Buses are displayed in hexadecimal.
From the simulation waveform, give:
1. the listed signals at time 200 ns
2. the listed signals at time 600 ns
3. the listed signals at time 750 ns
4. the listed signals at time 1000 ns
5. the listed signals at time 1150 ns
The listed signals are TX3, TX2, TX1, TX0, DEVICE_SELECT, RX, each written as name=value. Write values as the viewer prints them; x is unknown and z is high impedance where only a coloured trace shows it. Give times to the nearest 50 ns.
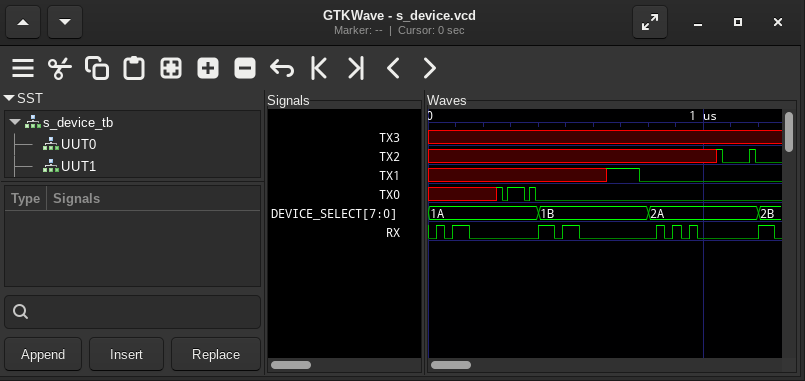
TX3=x, TX2=x, TX1=x, TX0=x, DEVICE_SELECT=1A, RX=0
TX3=x, TX2=x, TX1=x, TX0=0, DEVICE_SELECT=1B, RX=0
TX3=x, TX2=x, TX1=1, TX0=0, DEVICE_SELECT=1B, RX=0
TX3=x, TX2=x, TX1=0, TX0=0, DEVICE_SELECT=2A, RX=0
TX3=x, TX2=0, TX1=0, TX0=0, DEVICE_SELECT=2A, RX=0
